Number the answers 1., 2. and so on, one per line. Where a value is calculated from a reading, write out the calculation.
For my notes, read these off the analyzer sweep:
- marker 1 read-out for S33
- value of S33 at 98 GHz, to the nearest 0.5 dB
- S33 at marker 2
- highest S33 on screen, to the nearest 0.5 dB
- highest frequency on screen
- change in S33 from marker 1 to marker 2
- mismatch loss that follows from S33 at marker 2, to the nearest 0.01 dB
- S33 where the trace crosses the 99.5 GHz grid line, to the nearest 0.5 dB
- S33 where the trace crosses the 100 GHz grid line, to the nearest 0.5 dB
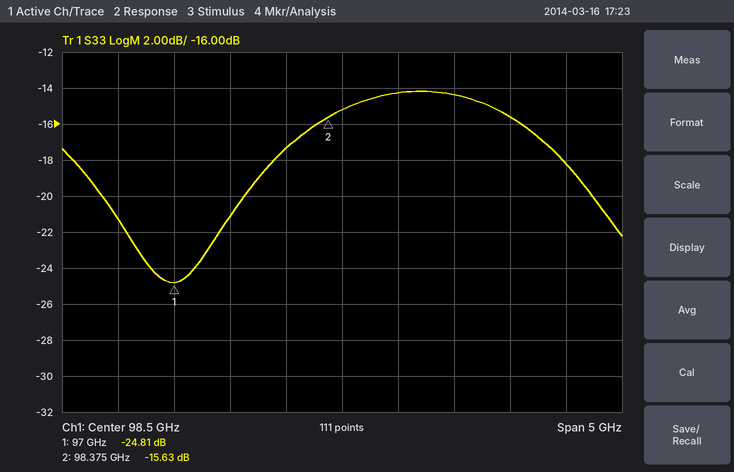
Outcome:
1. -24.81 dB
2. -17.5 dB
3. -15.63 dB
4. -14.0 dB
5. 101 GHz
6. -15.63 − (-24.81) = 9.18 dB
7. −10 log10(1 − 10^(-15.63/10)) ≈ 0.12 dB
8. -14.5 dB
9. -15.5 dB
